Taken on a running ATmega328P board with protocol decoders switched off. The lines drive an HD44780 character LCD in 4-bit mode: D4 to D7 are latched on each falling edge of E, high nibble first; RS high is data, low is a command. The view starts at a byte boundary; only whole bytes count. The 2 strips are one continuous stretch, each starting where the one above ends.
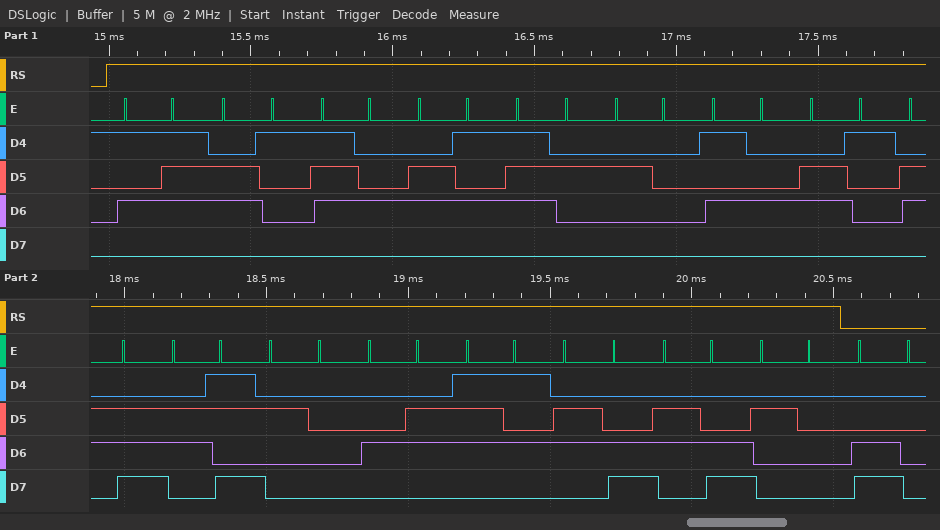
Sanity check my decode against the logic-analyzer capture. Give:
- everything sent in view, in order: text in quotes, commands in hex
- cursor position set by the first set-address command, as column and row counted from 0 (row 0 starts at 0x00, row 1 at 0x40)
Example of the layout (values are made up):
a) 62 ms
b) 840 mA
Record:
a) "Water Tank Full " 0xC0
b) column 0, row 1
